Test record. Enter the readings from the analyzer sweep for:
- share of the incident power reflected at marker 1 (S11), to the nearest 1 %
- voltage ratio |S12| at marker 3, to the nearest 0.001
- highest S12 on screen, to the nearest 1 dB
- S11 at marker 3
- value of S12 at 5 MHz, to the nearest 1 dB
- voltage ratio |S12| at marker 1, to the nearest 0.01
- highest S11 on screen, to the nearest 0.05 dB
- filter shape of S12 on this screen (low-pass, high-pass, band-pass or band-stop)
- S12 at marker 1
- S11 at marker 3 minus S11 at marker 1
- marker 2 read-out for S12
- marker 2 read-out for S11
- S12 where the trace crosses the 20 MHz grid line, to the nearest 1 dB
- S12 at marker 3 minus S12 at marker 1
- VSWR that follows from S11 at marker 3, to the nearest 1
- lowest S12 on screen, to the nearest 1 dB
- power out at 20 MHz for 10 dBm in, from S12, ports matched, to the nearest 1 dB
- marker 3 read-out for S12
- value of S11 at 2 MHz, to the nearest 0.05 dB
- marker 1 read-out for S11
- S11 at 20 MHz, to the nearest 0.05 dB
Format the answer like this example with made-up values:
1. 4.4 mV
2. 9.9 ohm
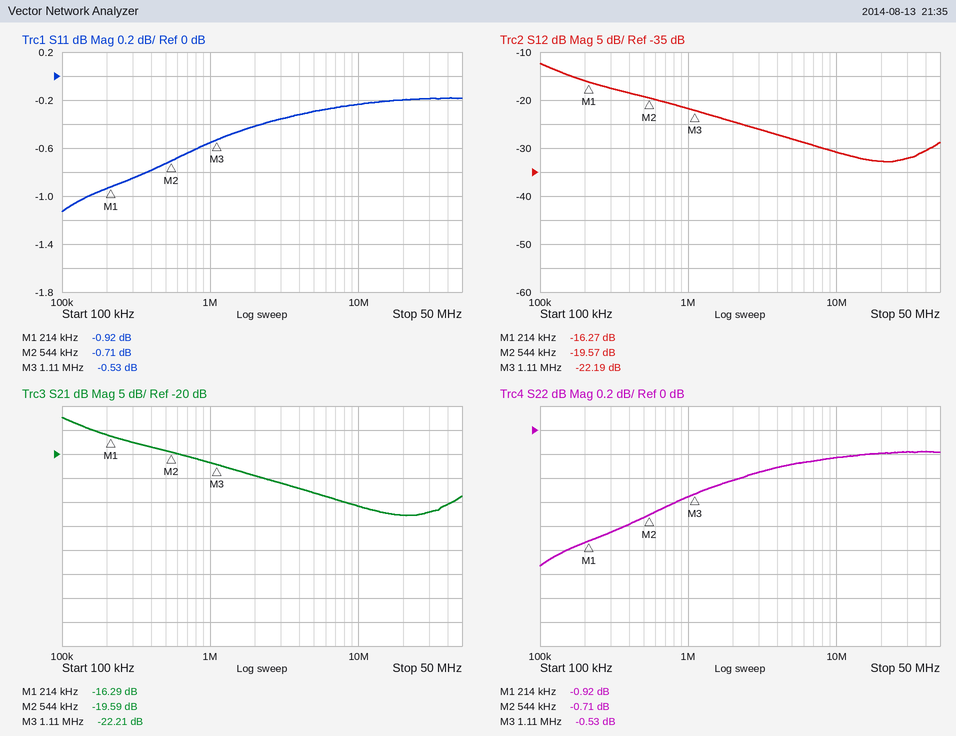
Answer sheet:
1. 81 %
2. 0.078
3. -12 dB
4. -0.53 dB
5. -28 dB
6. 0.15
7. -0.20 dB
8. low-pass
9. -16.27 dB
10. 0.39 dB
11. -19.57 dB
12. -0.71 dB
13. -33 dB
14. -5.92 dB
15. 33
16. -33 dB
17. -23 dBm
18. -22.19 dB
19. -0.40 dB
20. -0.92 dB
21. -0.20 dB
